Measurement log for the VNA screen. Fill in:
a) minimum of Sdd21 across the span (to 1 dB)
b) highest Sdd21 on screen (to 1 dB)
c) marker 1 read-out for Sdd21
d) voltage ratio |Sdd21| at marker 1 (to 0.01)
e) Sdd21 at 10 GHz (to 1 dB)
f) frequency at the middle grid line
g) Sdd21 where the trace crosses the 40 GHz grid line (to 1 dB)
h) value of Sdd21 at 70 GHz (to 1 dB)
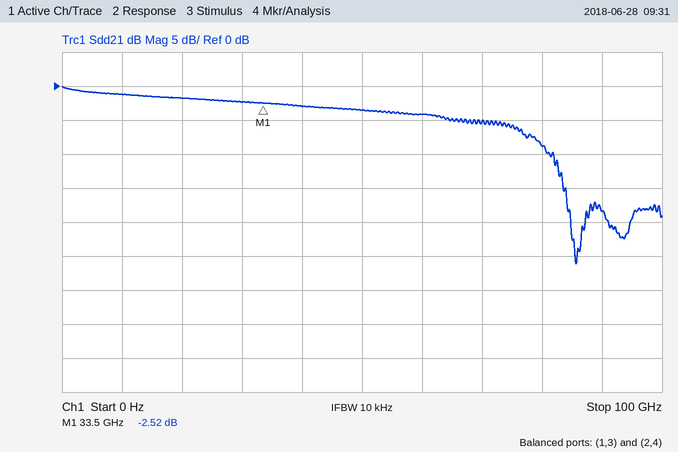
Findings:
-26 dB
0 dB
-2.52 dB
0.75
-1 dB
50 GHz
-3 dB
-5 dB
